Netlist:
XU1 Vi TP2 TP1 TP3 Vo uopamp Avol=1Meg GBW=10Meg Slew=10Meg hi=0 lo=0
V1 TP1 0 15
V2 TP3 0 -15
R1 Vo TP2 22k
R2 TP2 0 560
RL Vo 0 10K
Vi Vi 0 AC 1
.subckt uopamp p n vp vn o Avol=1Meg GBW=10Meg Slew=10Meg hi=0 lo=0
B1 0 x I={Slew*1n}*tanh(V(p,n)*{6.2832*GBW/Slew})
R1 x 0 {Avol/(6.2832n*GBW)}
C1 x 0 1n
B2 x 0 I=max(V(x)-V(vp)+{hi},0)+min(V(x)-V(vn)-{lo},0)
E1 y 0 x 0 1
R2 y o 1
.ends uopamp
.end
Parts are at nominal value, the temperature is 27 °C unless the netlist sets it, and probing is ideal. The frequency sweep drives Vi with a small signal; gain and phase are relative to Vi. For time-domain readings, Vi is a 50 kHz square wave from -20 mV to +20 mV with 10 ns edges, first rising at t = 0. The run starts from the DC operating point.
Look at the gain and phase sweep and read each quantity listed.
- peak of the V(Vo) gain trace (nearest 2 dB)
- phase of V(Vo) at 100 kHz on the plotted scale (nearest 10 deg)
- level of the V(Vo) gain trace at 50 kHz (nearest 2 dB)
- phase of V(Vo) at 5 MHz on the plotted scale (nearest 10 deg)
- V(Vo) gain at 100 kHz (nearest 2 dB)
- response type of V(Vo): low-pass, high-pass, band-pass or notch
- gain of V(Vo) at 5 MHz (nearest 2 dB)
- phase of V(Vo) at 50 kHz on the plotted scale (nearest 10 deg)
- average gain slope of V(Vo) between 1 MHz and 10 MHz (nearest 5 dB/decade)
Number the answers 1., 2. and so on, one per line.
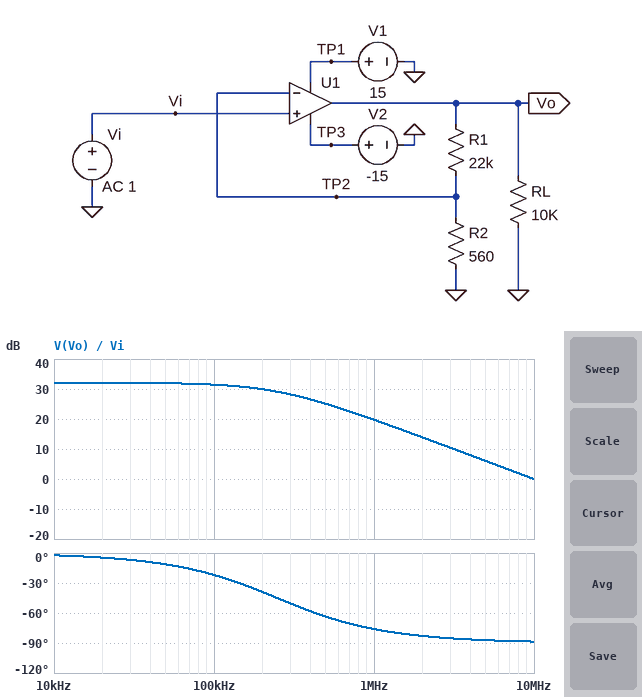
1. 32 dB
2. -20 deg
3. 32 dB
4. -90 deg
5. 32 dB
6. low-pass
7. 6 dB
8. -10 deg
9. -20 dB/decade
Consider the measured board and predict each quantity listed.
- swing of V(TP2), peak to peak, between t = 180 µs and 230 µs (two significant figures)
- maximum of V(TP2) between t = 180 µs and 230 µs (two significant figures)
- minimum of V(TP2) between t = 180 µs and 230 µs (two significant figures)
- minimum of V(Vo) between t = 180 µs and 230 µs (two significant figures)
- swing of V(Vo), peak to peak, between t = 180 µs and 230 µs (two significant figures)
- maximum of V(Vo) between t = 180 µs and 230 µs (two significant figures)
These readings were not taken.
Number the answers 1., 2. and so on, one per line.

1. 40 mV
2. 20 mV
3. -20 mV
4. -810 mV
5. 1.6 V
6. 810 mV
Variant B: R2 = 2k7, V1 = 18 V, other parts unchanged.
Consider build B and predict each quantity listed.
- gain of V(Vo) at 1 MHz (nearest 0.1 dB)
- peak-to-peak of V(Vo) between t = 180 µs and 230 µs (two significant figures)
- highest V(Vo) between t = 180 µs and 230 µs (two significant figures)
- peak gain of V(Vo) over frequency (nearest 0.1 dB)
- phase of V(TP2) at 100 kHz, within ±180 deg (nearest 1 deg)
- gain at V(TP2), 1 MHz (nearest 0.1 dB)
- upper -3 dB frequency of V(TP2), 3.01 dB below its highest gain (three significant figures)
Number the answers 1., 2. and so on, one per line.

1. 16.6 dB
2. 370 mV
3. 180 mV
4. 19.2 dB
5. -5 deg
6. -2.6 dB
7. 1.09 MHz
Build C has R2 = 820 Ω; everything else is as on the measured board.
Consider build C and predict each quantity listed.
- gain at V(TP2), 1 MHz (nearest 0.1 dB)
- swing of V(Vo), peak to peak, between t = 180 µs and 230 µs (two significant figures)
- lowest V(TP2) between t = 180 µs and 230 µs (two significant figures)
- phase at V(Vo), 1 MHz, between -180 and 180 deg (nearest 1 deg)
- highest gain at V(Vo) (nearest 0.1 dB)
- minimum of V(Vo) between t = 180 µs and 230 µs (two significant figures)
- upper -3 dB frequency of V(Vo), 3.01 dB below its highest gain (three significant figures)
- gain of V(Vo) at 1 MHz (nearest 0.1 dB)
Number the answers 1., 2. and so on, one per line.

1. -9.4 dB
2. 1.1 V
3. -20 mV
4. -70 deg
5. 28.9 dB
6. -560 mV
7. 359 kHz
8. 19.5 dB
